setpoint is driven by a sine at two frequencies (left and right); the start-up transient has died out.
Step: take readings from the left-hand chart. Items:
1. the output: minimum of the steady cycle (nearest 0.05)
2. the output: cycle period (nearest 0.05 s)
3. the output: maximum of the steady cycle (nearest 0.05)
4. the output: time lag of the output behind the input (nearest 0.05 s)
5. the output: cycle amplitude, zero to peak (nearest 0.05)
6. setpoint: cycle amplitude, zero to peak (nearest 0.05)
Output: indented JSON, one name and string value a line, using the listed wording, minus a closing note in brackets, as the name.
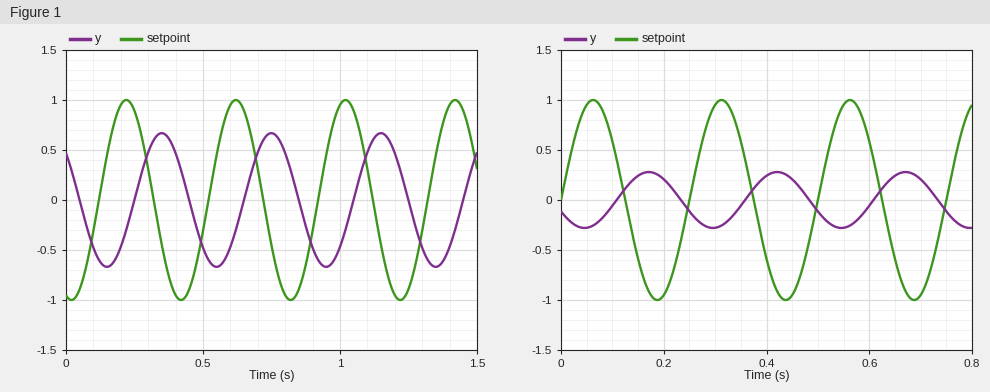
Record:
{
  "the output: minimum of the steady cycle": "-0.65",
  "the output: cycle period": "0.40 s",
  "the output: maximum of the steady cycle": "0.65",
  "the output: time lag of the output behind the input": "0.15 s",
  "the output: cycle amplitude, zero to peak": "0.65",
  "setpoint: cycle amplitude, zero to peak": "1.00"
}
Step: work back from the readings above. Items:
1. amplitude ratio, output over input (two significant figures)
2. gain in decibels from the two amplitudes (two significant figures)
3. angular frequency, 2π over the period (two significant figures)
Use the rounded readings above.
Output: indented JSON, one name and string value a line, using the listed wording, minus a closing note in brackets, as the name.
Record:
{
  "amplitude ratio, output over input": "0.65",
  "gain in decibels from the two amplitudes": "-3.7 dB",
  "angular frequency, 2π over the period": "16 rad/s"
}
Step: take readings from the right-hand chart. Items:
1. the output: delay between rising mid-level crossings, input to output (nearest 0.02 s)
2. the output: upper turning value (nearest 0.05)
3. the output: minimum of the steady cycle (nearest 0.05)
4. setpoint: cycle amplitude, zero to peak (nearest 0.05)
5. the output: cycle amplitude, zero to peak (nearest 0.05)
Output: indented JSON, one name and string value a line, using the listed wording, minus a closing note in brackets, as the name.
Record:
{
  "the output: delay between rising mid-level crossings, input to output": "0.10 s",
  "the output: upper turning value": "0.30",
  "the output: minimum of the steady cycle": "-0.30",
  "setpoint: cycle amplitude, zero to peak": "1.00",
  "the output: cycle amplitude, zero to peak": "0.30"
}
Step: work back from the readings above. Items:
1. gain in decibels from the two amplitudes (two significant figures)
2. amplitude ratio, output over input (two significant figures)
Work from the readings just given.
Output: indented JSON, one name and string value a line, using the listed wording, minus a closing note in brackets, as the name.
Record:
{
  "gain in decibels from the two amplitudes": "-10 dB",
  "amplitude ratio, output over input": "0.30"
}
